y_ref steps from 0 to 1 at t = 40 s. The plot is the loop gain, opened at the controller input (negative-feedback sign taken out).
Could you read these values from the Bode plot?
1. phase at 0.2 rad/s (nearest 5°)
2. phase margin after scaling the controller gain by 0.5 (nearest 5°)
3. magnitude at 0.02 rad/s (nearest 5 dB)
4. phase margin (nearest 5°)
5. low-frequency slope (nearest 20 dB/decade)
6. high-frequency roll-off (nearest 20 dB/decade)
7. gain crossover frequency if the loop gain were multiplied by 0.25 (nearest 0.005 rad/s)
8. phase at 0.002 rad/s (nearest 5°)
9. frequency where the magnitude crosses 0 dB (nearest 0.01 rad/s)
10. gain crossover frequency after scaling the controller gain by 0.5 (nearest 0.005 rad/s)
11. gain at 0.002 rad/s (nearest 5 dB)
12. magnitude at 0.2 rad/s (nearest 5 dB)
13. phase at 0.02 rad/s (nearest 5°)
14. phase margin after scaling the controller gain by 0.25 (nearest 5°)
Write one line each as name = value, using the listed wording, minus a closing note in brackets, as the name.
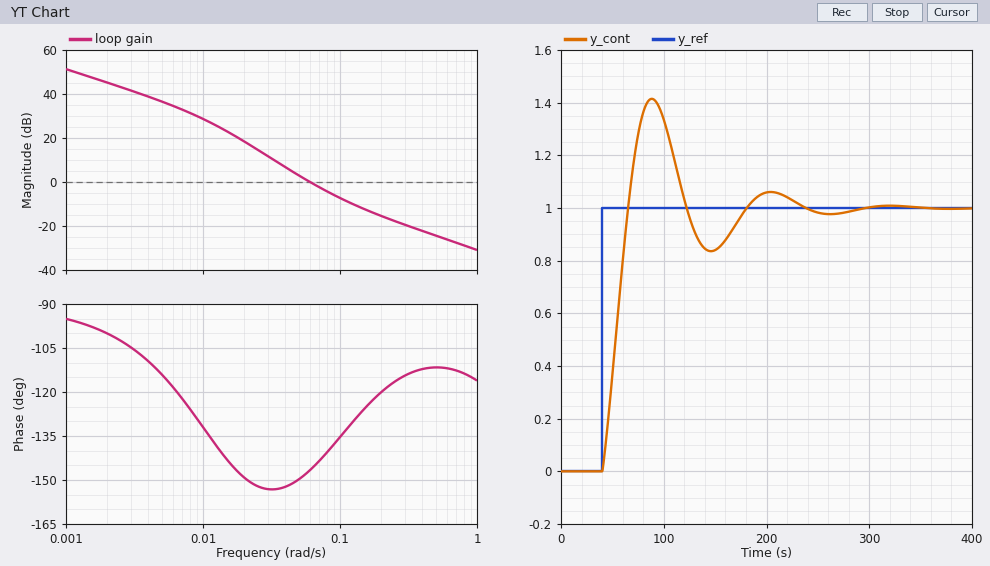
phase at 0.2 rad/s = -120°
phase margin after scaling the controller gain by 0.5 = 30°
magnitude at 0.02 rad/s = 20 dB
phase margin = 35°
low-frequency slope = -20 dB/decade
high-frequency roll-off = -20 dB/decade
gain crossover frequency if the loop gain were multiplied by 0.25 = 0.030 rad/s
phase at 0.002 rad/s = -100°
frequency where the magnitude crosses 0 dB = 0.06 rad/s
gain crossover frequency after scaling the controller gain by 0.5 = 0.040 rad/s
gain at 0.002 rad/s = 45 dB
magnitude at 0.2 rad/s = -15 dB
phase at 0.02 rad/s = -150°
phase margin after scaling the controller gain by 0.25 = 25°
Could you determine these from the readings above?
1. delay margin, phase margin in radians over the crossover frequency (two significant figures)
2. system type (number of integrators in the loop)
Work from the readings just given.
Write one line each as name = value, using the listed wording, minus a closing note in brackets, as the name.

delay margin, phase margin in radians over the crossover frequency = 10 s
system type = 1
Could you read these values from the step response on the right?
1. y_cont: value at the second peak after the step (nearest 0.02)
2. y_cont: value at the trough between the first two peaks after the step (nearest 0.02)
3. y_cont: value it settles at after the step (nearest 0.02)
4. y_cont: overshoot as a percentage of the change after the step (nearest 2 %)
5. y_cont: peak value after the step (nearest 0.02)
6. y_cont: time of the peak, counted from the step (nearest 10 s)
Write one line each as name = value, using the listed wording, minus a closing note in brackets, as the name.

y_cont: value at the second peak after the step = 1.06
y_cont: value at the trough between the first two peaks after the step = 0.84
y_cont: value it settles at after the step = 1.00
y_cont: overshoot as a percentage of the change after the step = 42 %
y_cont: peak value after the step = 1.42
y_cont: time of the peak, counted from the step = 50 s
